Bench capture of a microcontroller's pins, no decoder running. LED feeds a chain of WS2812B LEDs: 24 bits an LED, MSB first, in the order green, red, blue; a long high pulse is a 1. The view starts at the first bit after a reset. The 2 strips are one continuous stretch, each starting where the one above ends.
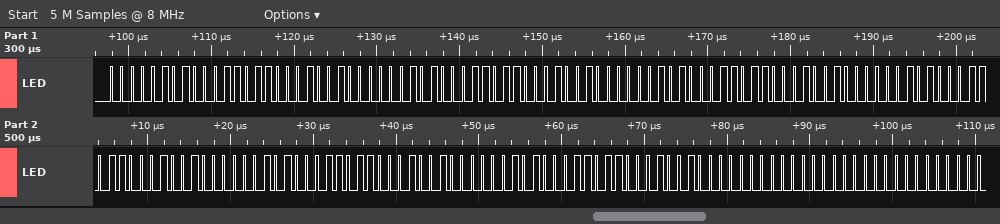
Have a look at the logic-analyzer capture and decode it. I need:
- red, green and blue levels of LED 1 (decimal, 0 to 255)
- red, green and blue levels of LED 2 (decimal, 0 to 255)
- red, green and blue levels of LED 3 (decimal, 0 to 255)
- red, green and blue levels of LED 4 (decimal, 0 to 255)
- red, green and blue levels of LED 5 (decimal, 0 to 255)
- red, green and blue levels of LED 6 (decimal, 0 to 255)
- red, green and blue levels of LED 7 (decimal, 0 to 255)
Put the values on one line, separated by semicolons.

27, 5, 18; 27, 5, 18; 27, 5, 18; 27, 5, 18; 27, 5, 18; 27, 5, 18; 0, 0, 0
